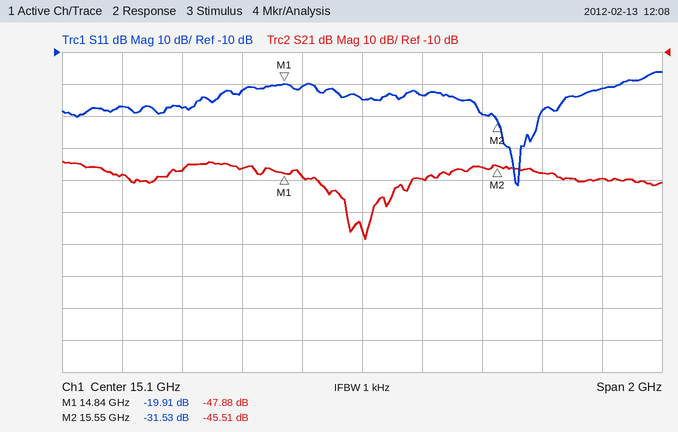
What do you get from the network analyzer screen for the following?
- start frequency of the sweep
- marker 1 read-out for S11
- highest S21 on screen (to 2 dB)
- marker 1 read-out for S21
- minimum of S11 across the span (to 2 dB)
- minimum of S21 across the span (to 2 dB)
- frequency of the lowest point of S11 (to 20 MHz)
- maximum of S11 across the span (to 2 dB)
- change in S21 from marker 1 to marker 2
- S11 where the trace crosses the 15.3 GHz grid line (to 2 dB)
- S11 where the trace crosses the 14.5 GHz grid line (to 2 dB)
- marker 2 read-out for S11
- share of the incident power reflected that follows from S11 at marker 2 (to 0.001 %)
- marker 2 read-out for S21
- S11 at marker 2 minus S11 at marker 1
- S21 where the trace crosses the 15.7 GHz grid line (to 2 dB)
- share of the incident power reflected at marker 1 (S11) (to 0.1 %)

14.1 GHz
-19.91 dB
-44 dB
-47.88 dB
-52 dB
-68 dB
15.62 GHz
-16 dB
2.37 dB
-24 dB
-28 dB
-31.53 dB
0.070 %
-45.51 dB
-11.62 dB
-48 dB
1.0 %
